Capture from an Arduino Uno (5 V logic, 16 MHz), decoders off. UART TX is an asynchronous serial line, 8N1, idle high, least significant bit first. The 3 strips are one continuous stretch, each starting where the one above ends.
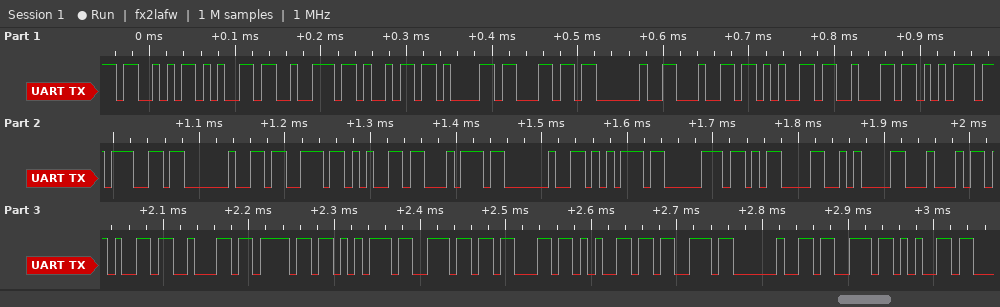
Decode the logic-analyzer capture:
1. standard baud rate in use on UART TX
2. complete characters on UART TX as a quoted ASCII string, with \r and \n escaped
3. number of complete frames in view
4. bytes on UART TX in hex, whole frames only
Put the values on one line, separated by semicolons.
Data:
115200 baud; "Serial debug set up\r\nDebounces se"; 33; 53 65 72 69 61 6C 20 64 65 62 75 67 20 73 65 74 20 75 70 0D 0A 44 65 62 6F 75 6E 63 65 73 20 73 65
